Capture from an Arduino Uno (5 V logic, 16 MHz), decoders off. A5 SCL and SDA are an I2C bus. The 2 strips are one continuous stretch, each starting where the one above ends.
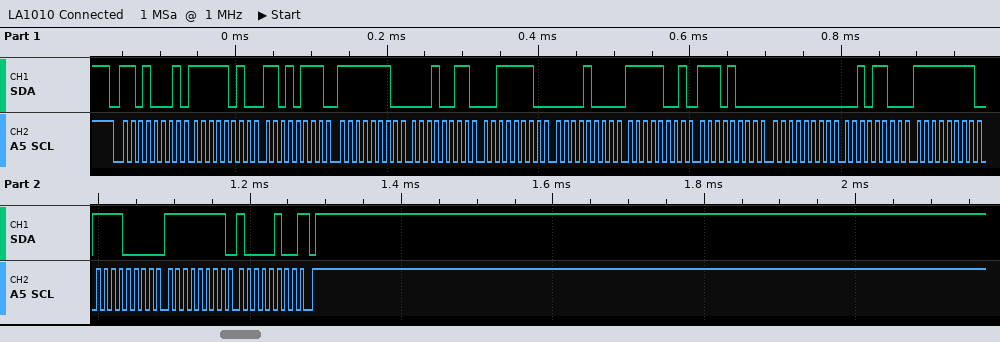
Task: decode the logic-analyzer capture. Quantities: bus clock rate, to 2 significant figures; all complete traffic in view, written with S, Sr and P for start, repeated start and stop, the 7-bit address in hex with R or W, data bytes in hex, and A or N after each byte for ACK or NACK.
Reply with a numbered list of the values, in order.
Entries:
1. 100 kHz
2. S 68R A FA A D7 A FE A 13 A 3E A 08 A F9 A E8 A 00 A 2C A FF A F0 A FF A 84 N P
